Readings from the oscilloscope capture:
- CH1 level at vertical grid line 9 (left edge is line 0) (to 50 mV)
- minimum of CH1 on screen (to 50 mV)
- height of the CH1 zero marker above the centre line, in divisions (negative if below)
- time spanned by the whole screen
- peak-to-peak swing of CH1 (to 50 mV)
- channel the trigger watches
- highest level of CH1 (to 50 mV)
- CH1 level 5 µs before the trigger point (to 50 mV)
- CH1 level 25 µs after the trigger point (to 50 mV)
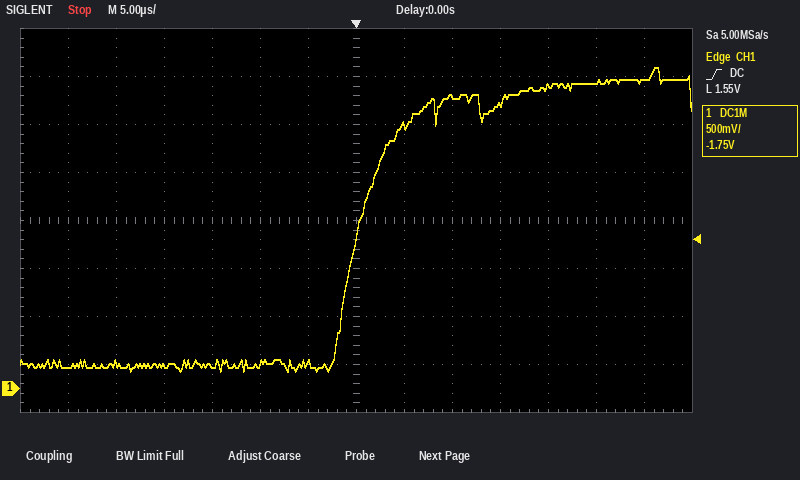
3.05 V
200 mV
-3.5 div
70 µs
3.15 V
CH1
3.35 V
250 mV
3.20 V
